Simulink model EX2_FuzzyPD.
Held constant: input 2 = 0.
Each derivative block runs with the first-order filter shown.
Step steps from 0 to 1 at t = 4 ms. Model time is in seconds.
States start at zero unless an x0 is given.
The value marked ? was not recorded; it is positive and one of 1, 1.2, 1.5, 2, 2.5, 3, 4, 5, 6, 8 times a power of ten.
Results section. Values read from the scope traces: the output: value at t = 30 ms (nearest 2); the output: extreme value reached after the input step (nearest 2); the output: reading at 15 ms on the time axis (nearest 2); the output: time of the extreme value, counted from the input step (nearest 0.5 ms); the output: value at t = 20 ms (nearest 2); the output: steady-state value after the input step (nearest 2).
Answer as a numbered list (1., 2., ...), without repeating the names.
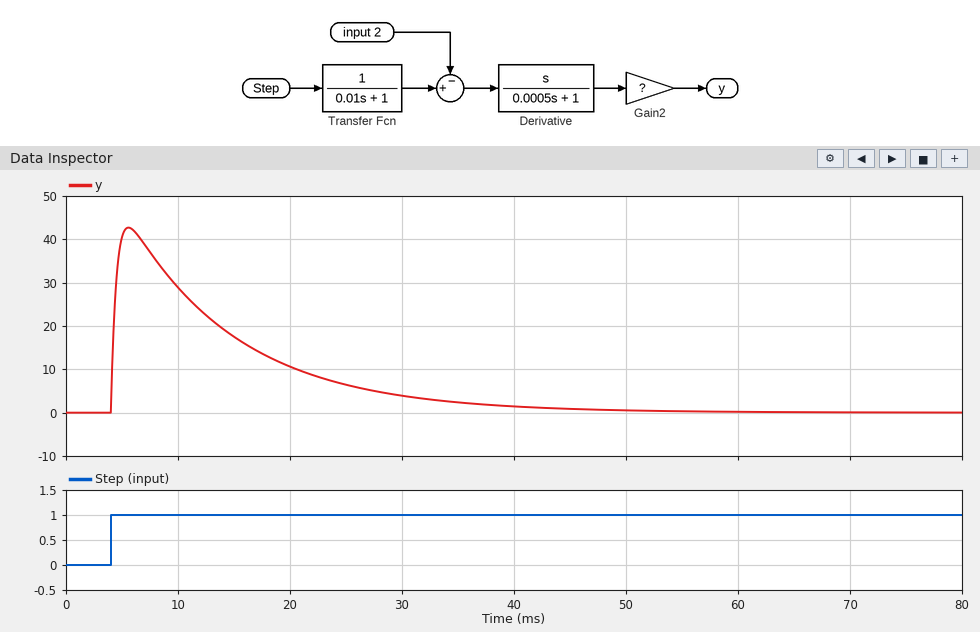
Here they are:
1. 4
2. 42
3. 18
4. 1.5 ms
5. 10
6. 0
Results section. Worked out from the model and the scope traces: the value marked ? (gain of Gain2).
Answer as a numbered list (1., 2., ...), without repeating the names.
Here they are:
1. 0.5
